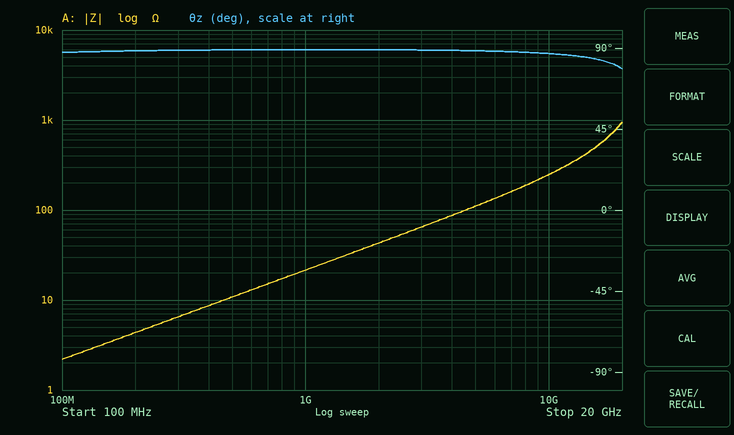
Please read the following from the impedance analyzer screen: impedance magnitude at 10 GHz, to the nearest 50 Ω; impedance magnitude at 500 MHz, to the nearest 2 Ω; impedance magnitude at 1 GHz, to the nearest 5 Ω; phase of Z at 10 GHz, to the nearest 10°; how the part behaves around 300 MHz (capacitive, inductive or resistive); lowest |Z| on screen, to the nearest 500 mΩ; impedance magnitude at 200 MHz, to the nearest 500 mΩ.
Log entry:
250 Ω
10 Ω
20 Ω
90°
inductive
2.0 Ω
4.5 Ω
